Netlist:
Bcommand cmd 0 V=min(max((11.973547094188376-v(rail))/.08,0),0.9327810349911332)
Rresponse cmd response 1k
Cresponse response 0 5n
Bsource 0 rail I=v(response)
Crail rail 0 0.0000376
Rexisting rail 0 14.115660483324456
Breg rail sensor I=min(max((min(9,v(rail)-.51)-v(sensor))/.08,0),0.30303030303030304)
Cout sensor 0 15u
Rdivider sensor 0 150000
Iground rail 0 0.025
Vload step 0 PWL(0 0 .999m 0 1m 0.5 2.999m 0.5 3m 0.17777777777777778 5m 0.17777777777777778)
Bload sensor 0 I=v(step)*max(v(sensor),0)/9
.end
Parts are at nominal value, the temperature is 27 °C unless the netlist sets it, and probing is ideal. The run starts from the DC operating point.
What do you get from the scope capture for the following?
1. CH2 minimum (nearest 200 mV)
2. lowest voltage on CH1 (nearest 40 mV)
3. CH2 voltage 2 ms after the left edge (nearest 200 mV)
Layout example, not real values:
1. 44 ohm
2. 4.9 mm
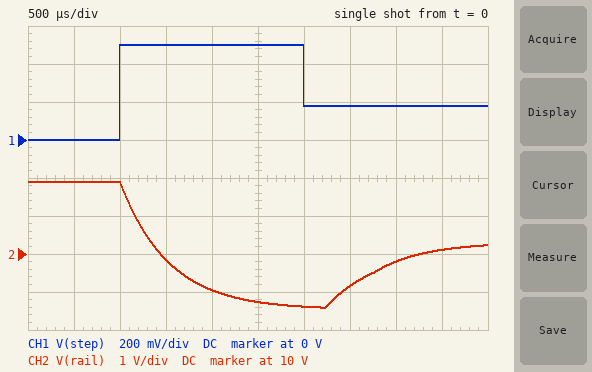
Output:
1. 8.6 V
2. 0 V
3. 9.0 V
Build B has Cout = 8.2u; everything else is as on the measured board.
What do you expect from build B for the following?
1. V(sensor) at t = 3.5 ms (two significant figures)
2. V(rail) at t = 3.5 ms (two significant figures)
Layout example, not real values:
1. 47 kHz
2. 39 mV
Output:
1. 8.9 V
2. 9.4 V
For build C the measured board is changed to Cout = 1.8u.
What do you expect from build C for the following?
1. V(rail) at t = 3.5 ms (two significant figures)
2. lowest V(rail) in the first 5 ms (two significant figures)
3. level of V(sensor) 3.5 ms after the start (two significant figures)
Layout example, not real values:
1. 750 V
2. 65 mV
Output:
1. 9.6 V
2. 8.6 V
3. 9.0 V
